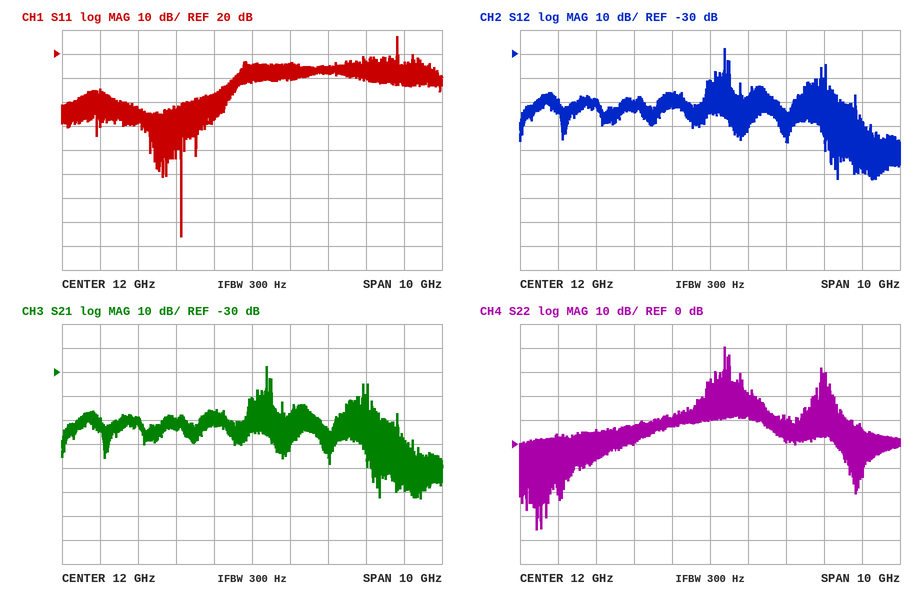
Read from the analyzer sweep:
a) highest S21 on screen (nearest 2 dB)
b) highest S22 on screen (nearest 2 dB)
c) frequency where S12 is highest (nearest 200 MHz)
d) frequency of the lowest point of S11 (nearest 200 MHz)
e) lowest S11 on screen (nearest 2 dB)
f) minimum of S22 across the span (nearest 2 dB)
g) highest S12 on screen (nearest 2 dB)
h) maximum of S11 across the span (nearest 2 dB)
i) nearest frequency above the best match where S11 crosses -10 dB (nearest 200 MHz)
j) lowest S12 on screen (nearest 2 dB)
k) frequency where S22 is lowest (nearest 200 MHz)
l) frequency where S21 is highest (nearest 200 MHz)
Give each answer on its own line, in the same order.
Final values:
-28 dB
40 dB
12.4 GHz
10.2 GHz
-56 dB
-36 dB
-28 dB
28 dB
10.2 GHz
-82 dB
7.4 GHz
12.4 GHz
